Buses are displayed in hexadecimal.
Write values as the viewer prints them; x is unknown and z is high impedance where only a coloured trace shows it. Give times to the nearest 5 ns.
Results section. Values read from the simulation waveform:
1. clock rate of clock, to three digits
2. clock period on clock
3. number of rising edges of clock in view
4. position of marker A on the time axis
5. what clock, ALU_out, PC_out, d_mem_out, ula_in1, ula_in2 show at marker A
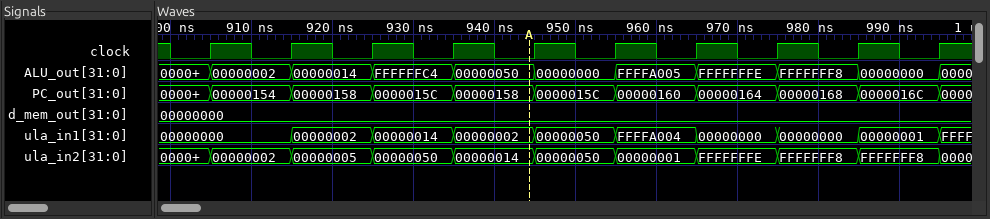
100 MHz
10 ns
10
945 ns
clock=0, ALU_out=00000050, PC_out=00000158, d_mem_out=00000000, ula_in1=00000002, ula_in2=00000014
